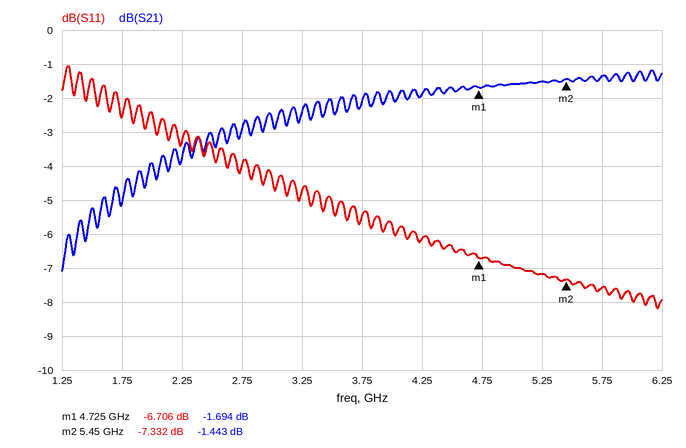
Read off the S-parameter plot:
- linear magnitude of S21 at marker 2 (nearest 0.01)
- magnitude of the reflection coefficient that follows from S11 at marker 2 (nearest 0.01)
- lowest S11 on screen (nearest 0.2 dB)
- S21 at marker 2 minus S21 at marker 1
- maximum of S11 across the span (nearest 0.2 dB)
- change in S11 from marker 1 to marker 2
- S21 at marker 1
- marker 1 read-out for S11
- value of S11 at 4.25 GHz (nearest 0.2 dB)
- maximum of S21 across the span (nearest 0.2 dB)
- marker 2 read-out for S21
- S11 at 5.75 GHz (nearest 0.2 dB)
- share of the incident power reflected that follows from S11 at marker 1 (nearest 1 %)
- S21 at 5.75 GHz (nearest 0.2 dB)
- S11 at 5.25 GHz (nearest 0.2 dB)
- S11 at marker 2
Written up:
0.85
0.43
-8.2 dB
0.251 dB
-1.0 dB
-0.626 dB
-1.694 dB
-6.706 dB
-6.2 dB
-1.2 dB
-1.443 dB
-7.6 dB
21 %
-1.4 dB
-7.2 dB
-7.332 dB
